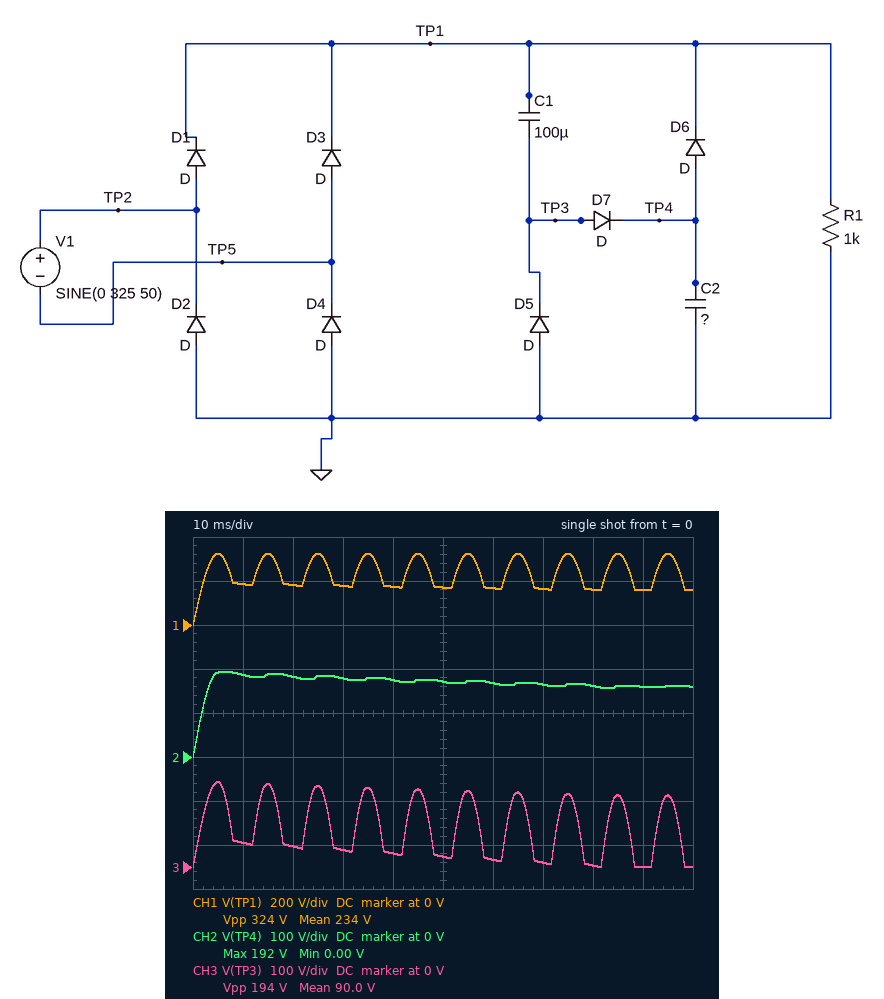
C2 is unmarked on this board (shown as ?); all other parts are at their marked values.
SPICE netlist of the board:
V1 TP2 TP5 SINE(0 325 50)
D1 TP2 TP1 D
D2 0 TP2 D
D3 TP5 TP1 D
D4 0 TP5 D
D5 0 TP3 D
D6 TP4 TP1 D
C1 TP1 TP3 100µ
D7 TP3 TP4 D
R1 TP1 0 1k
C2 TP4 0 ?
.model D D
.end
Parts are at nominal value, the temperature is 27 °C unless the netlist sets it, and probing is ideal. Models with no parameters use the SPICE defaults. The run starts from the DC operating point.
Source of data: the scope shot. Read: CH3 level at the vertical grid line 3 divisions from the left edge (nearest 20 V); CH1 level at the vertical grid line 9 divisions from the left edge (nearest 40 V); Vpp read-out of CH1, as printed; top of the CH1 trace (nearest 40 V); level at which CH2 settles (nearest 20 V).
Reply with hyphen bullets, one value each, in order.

- 40 V
- 160 V
- 324 V
- 320 V
- 160 V
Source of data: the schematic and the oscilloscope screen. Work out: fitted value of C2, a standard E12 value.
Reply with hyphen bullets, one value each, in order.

- 68 µF
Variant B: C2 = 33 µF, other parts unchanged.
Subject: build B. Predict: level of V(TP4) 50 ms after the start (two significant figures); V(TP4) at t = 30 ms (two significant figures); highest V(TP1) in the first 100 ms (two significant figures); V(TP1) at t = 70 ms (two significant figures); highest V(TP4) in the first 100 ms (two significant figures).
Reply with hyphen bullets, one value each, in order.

- 200 V
- 210 V
- 320 V
- 190 V
- 240 V
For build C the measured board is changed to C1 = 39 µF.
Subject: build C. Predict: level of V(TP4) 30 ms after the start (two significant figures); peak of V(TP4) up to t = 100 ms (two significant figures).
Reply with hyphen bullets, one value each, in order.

- 130 V
- 160 V
